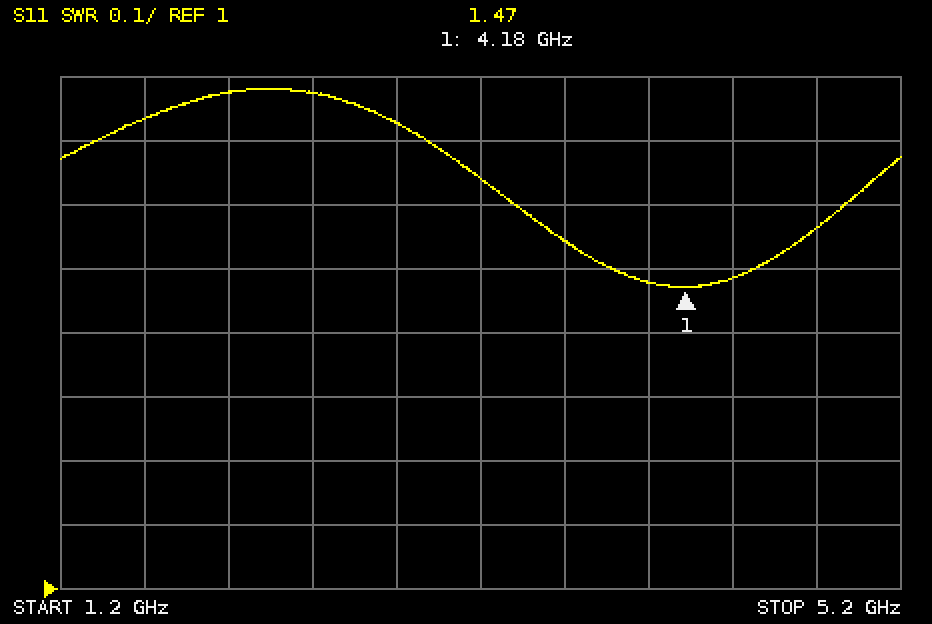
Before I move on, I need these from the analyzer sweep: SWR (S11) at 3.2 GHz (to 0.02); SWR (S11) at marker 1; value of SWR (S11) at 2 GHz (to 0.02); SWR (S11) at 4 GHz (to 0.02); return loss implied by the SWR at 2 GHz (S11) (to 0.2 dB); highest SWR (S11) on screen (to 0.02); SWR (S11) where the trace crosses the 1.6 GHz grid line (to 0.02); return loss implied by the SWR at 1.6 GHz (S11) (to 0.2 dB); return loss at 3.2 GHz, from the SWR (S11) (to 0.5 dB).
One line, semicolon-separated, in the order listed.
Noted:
1.64; 1.47; 1.78; 1.48; 11.0 dB; 1.78; 1.74; 11.4 dB; 12.5 dB
